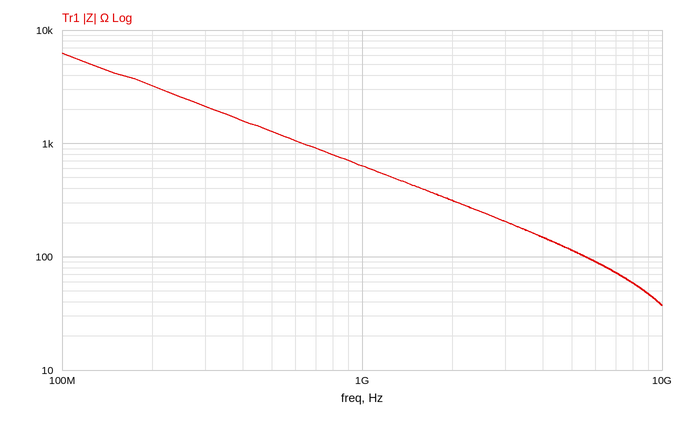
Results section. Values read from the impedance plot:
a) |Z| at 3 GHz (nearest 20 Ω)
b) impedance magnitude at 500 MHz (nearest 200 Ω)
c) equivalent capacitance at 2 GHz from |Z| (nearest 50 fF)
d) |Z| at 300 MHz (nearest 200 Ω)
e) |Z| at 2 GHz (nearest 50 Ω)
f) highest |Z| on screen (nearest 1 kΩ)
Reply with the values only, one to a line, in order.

200 Ω
1.2 kΩ
250 fF
2.2 kΩ
300 Ω
6 kΩ
